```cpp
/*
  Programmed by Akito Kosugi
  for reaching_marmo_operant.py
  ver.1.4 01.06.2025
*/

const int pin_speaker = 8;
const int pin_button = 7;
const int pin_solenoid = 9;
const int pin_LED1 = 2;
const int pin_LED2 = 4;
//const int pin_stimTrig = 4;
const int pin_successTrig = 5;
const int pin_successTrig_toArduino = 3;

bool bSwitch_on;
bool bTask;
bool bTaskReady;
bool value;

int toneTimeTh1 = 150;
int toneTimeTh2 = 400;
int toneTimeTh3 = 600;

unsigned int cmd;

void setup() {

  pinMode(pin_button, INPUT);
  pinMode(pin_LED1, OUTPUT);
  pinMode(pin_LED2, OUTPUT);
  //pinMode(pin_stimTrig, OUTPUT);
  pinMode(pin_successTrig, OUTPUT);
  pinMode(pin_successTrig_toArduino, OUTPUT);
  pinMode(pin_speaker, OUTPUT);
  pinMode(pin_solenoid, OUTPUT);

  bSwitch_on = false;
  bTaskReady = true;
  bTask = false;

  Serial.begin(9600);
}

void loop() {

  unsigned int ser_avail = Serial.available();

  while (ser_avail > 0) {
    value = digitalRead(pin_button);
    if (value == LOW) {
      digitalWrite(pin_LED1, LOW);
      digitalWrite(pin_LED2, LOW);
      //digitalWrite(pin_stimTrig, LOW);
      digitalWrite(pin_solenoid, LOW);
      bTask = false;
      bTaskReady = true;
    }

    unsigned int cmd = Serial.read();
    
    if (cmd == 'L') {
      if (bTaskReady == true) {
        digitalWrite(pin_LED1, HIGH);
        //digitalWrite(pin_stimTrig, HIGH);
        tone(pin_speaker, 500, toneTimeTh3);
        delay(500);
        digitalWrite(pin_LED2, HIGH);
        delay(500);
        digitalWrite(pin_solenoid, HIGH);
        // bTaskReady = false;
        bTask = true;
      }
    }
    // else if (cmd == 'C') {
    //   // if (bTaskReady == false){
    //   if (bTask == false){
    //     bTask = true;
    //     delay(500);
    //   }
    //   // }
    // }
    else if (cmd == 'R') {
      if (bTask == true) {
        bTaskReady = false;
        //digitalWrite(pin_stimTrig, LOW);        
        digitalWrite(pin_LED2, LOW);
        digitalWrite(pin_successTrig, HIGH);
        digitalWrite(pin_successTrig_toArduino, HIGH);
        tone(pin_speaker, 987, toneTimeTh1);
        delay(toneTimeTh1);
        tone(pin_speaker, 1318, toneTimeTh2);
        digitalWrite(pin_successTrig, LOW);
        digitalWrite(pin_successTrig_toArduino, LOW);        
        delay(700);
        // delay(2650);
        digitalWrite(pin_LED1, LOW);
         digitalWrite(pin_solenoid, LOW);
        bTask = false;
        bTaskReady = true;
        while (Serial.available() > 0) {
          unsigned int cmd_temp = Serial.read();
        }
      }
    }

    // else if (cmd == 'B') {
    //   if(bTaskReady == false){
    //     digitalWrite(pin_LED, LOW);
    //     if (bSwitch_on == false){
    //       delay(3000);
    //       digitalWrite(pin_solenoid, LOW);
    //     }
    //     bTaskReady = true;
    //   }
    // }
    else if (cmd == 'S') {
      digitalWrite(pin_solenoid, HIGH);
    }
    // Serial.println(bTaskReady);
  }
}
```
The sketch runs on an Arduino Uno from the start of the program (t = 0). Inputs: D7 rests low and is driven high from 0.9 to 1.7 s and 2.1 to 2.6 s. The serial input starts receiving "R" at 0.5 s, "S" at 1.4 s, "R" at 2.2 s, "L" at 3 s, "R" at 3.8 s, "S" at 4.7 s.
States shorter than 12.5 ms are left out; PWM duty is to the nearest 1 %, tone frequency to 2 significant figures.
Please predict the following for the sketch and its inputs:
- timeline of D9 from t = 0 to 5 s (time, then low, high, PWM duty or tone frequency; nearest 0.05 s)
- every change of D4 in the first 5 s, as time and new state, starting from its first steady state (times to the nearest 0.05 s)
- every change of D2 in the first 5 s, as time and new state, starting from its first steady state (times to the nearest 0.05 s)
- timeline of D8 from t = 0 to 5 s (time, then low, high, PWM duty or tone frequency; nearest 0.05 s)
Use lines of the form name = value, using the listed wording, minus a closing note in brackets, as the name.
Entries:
timeline of D9 from t = 0 to 5 s = 0 s low; 1.4 s high; 1.7 s low
every change of D4 in the first 5 s, as time and new state, starting from its first steady state = 0 s low; 3.5 s high; 4 s low
every change of D2 in the first 5 s, as time and new state, starting from its first steady state = 0 s low; 3 s high; 4 s low
timeline of D8 from t = 0 to 5 s = 0 s low; 3 s tone 500 Hz; 3.6 s low
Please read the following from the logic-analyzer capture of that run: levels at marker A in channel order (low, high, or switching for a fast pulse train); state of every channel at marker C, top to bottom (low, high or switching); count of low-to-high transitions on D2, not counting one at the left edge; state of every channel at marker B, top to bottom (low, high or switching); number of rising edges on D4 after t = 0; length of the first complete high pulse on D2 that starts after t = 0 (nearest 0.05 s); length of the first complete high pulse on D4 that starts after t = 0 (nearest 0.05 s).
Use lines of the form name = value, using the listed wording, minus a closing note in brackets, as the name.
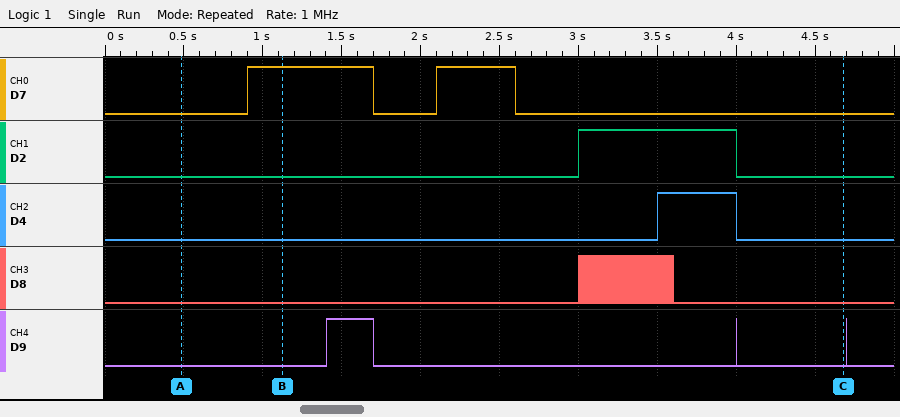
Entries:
levels at marker A in channel order = D7 low, D2 low, D4 low, D8 low, D9 low
state of every channel at marker C, top to bottom = D7 low, D2 low, D4 low, D8 low, D9 low
count of low-to-high transitions on D2, not counting one at the left edge = 1
state of every channel at marker B, top to bottom = D7 high, D2 low, D4 low, D8 low, D9 low
number of rising edges on D4 after t = 0 = 1
length of the first complete high pulse on D2 that starts after t = 0 = 1.00 s
length of the first complete high pulse on D4 that starts after t = 0 = 0.50 s
